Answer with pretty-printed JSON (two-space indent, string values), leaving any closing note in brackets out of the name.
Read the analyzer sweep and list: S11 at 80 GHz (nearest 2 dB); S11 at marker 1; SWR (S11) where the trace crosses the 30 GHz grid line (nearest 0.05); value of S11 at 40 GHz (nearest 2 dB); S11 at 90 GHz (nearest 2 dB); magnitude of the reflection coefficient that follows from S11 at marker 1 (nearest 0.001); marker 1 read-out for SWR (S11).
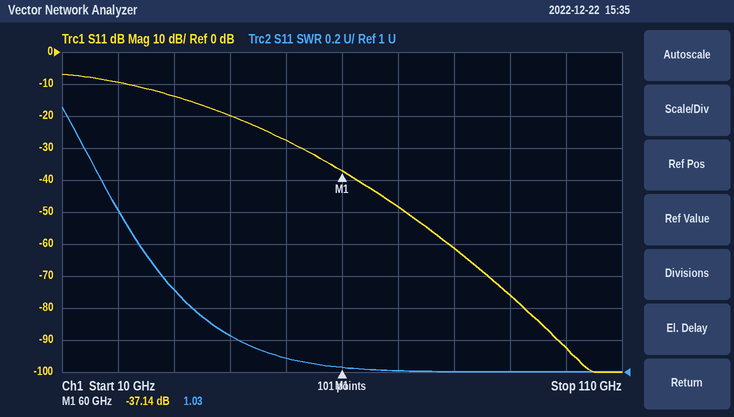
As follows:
{
  "S11 at 80 GHz": "-62 dB",
  "S11 at marker 1": "-37.14 dB",
  "SWR (S11) where the trace crosses the 30 GHz grid line": "1.50",
  "value of S11 at 40 GHz": "-20 dB",
  "S11 at 90 GHz": "-76 dB",
  "magnitude of the reflection coefficient that follows from S11 at marker 1": "0.014",
  "marker 1 read-out for SWR": "1.03"
}
